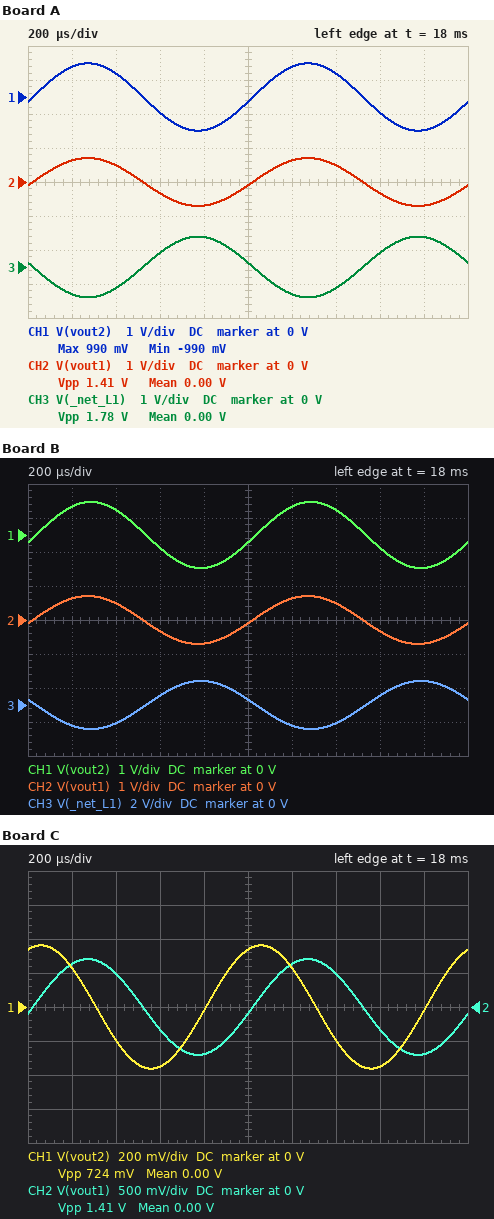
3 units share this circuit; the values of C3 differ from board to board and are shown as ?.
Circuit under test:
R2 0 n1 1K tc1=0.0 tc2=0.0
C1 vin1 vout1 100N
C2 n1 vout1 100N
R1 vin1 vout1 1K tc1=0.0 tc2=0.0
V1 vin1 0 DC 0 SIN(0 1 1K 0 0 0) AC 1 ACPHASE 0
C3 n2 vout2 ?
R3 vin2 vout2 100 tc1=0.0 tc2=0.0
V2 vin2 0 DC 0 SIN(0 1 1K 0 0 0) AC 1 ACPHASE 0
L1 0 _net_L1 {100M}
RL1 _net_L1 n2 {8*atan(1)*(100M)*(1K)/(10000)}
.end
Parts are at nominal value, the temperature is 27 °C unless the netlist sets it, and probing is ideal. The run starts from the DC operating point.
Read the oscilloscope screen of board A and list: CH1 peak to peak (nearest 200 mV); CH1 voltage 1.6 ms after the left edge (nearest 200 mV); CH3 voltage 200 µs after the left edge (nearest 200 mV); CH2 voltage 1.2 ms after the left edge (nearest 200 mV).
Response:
2.0 V
-400 mV
-800 mV
600 mV
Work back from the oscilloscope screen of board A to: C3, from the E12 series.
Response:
120 nF
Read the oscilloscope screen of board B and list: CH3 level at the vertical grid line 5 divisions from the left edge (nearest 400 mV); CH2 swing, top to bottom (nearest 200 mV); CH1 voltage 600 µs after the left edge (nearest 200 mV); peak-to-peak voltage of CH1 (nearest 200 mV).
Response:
400 mV
1.4 V
-400 mV
2.0 V
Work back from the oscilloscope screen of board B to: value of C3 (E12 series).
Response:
150 nF
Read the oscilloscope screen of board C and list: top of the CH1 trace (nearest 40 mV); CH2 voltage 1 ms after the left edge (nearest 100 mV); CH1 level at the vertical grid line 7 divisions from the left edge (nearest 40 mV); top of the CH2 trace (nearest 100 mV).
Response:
360 mV
-100 mV
-200 mV
700 mV
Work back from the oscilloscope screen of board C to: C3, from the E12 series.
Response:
270 nF
